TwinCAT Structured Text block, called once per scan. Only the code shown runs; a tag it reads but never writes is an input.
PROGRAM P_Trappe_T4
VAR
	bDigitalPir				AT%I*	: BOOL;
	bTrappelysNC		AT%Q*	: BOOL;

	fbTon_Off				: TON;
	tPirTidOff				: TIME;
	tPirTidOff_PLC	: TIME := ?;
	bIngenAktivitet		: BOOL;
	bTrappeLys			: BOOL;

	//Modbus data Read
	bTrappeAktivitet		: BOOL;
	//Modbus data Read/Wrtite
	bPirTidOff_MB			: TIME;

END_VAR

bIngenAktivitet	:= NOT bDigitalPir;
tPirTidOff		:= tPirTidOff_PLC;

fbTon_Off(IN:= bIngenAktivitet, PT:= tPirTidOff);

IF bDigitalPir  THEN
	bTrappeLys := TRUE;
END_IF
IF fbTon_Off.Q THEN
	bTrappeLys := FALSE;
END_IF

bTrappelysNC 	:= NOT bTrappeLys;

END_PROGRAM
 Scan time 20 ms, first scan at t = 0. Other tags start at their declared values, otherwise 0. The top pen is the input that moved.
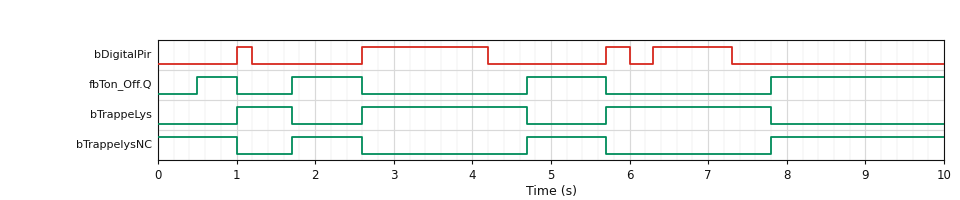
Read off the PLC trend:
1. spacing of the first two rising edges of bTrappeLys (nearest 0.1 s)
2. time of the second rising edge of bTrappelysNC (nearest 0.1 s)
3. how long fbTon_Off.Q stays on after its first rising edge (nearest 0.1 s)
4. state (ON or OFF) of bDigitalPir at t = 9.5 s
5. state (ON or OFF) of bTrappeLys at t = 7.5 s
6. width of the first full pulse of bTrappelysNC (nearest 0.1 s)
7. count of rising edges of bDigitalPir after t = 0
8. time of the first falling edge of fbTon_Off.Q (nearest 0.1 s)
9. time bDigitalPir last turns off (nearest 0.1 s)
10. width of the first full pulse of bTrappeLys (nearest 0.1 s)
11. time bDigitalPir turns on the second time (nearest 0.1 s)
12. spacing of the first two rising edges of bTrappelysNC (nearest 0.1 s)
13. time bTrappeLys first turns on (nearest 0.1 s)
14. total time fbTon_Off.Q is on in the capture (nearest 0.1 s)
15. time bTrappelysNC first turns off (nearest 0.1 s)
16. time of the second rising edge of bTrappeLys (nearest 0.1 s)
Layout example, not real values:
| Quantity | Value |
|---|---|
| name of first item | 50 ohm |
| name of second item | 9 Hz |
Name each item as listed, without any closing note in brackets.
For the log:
| Quantity | Value |
|---|---|
| spacing of the first two rising edges of bTrappeLys | 1.6 s |
| time of the second rising edge of bTrappelysNC | 4.7 s |
| how long fbTon_Off.Q stays on after its first rising edge | 0.5 s |
| state (ON or OFF) of bDigitalPir at t = 9.5 s | OFF |
| state (ON or OFF) of bTrappeLys at t = 7.5 s | ON |
| width of the first full pulse of bTrappelysNC | 0.9 s |
| count of rising edges of bDigitalPir after t = 0 | 4 |
| time of the first falling edge of fbTon_Off.Q | 1.0 s |
| time bDigitalPir last turns off | 7.3 s |
| width of the first full pulse of bTrappeLys | 0.7 s |
| time bDigitalPir turns on the second time | 2.6 s |
| spacing of the first two rising edges of bTrappelysNC | 3.0 s |
| time bTrappeLys first turns on | 1.0 s |
| total time fbTon_Off.Q is on in the capture | 4.6 s |
| time bTrappelysNC first turns off | 1.0 s |
| time of the second rising edge of bTrappeLys | 2.6 s |
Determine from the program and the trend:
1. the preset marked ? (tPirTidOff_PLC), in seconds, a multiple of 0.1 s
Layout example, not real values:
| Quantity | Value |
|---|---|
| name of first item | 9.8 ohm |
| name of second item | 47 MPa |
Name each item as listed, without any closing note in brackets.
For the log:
| Quantity | Value |
|---|---|
| the preset marked ? (tPirTidOff_PLC), in seconds, a multiple of 0.1 s | 0.5 s |
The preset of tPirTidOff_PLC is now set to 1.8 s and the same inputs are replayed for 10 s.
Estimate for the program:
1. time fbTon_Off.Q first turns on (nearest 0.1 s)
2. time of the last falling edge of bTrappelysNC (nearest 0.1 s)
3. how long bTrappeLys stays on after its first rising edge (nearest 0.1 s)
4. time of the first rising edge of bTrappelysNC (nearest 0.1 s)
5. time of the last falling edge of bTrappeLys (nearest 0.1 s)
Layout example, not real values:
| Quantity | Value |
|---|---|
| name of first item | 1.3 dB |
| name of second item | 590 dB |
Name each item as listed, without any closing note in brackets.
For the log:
| Quantity | Value |
|---|---|
| time fbTon_Off.Q first turns on | 9.1 s |
| time of the last falling edge of bTrappelysNC | 1.0 s |
| how long bTrappeLys stays on after its first rising edge | 8.1 s |
| time of the first rising edge of bTrappelysNC | 9.1 s |
| time of the last falling edge of bTrappeLys | 9.1 s |
